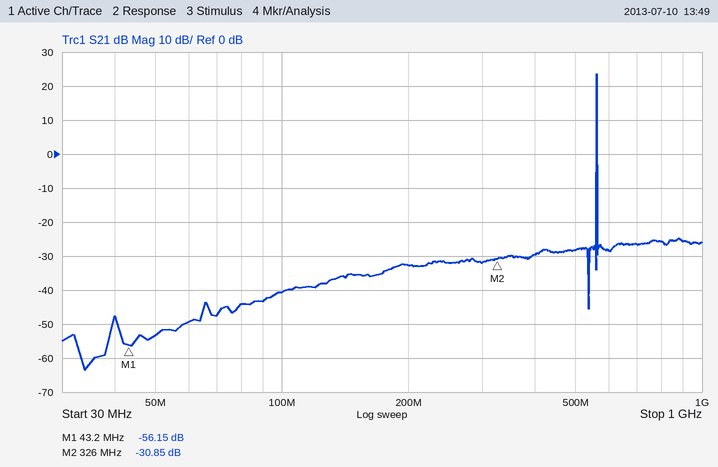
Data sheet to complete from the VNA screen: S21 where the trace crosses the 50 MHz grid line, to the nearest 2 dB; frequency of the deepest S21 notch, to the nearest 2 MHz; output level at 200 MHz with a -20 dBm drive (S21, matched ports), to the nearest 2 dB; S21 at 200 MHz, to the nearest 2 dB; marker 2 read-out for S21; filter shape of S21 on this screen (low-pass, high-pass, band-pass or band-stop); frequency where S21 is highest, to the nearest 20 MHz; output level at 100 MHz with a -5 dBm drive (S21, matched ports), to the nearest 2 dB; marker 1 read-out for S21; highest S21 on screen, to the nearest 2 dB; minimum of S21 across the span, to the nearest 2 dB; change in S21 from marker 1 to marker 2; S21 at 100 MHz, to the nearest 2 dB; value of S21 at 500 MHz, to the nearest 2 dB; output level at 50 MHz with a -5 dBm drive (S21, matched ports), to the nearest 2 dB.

-54 dB
34 MHz
-52 dBm
-32 dB
-30.85 dB
band-pass
560 MHz
-46 dBm
-56.15 dB
24 dB
-64 dB
25.30 dB
-40 dB
-28 dB
-58 dBm
